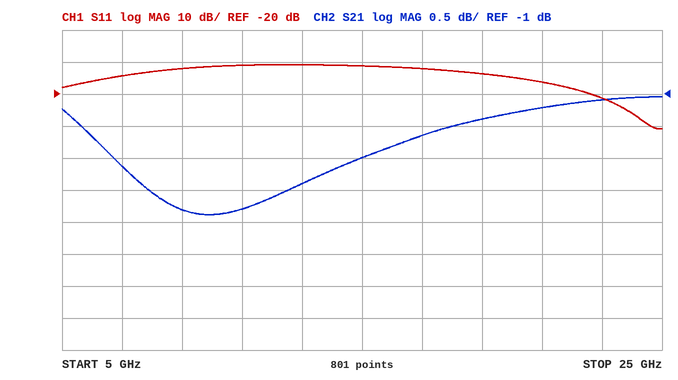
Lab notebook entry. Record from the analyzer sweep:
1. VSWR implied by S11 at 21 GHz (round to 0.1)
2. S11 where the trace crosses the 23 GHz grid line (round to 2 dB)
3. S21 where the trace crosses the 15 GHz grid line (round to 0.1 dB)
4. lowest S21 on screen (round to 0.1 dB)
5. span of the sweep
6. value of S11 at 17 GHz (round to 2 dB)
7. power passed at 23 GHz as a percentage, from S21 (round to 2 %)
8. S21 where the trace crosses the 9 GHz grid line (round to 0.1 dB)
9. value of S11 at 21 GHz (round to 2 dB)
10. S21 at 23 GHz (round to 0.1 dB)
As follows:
1.4
-22 dB
-2.0 dB
-2.9 dB
20 GHz
-12 dB
78 %
-2.8 dB
-16 dB
-1.1 dB
